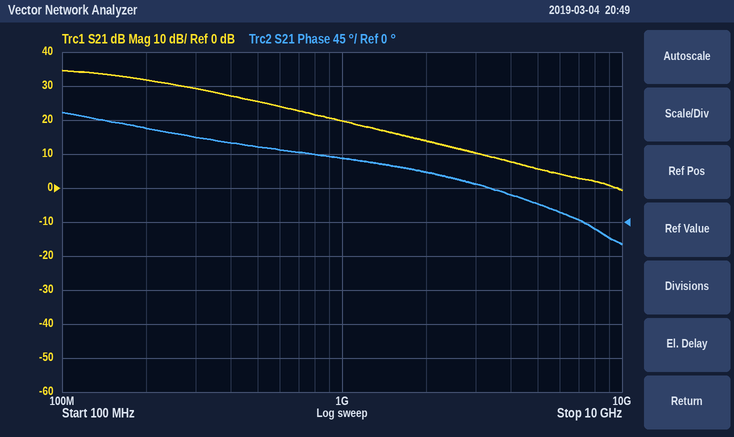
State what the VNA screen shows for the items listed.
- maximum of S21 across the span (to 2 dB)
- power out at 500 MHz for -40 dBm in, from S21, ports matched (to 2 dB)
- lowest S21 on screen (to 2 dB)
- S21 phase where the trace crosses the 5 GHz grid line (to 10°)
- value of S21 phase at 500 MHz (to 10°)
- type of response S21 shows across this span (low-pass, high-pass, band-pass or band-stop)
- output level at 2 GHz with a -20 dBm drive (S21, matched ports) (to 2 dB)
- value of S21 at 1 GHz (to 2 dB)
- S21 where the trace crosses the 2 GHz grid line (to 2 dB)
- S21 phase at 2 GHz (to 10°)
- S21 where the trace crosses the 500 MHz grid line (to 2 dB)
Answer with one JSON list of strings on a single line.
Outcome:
["34 dB", "-14 dBm", "0 dB", "20°", "100°", "low-pass", "-6 dBm", "20 dB", "14 dB", "70°", "26 dB"]
